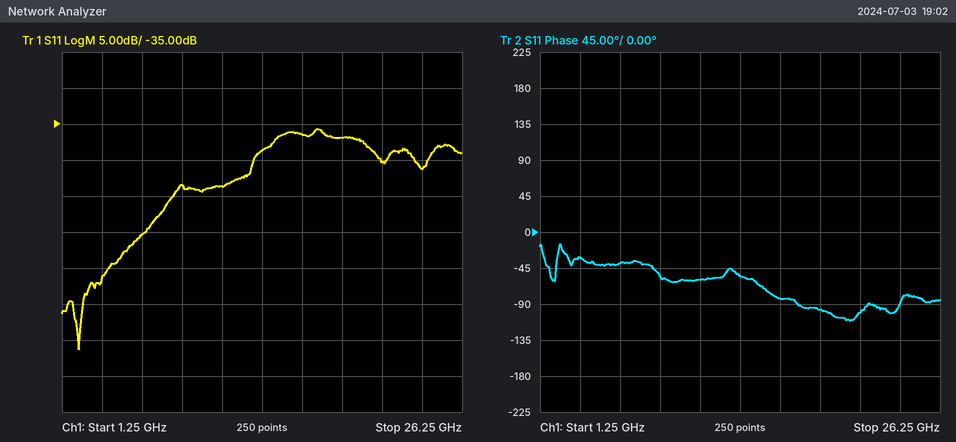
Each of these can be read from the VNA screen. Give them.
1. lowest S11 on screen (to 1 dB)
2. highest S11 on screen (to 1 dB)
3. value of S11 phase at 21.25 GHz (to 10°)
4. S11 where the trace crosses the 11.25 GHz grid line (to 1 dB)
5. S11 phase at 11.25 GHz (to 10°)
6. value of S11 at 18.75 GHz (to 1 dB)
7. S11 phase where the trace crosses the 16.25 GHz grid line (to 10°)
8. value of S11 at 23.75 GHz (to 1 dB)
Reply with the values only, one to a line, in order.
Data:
-66 dB
-36 dB
-100°
-44 dB
-60°
-37 dB
-80°
-41 dB
